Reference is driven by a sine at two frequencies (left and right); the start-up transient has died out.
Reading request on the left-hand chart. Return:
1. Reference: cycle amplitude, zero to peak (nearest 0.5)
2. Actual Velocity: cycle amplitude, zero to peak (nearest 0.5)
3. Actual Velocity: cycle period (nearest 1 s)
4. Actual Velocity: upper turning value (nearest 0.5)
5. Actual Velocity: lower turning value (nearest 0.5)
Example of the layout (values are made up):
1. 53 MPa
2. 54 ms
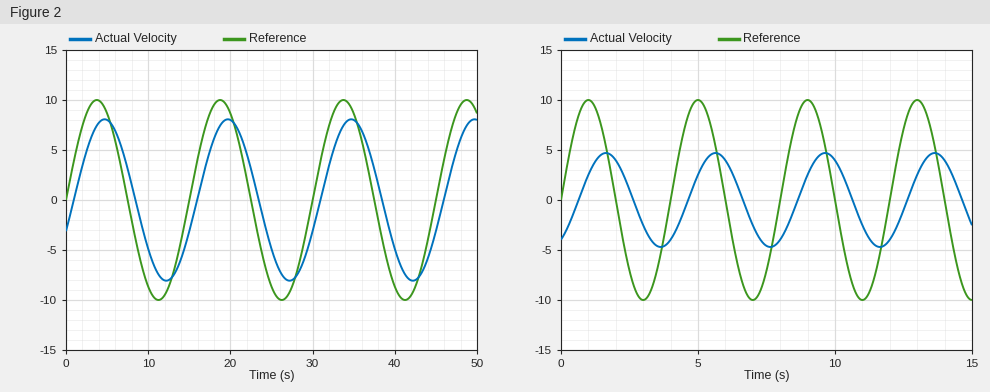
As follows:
1. 10.0
2. 8.0
3. 15 s
4. 8.0
5. -8.0
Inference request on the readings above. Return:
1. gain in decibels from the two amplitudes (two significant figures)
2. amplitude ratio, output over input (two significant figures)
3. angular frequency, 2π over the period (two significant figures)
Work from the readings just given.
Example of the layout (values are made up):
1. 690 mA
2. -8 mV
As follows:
1. -1.9 dB
2. 0.80
3. 0.42 rad/s
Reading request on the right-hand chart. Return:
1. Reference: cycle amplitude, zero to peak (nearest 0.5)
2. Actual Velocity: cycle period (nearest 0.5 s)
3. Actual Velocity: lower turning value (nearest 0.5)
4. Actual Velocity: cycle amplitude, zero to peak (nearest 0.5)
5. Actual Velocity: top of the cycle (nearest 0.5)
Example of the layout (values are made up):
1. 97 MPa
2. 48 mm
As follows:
1. 10.0
2. 4.0 s
3. -4.5
4. 4.5
5. 4.5
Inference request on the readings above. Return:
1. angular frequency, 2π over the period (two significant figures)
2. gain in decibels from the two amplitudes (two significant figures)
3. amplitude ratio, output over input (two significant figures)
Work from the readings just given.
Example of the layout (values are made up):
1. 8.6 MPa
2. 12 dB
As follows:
1. 1.6 rad/s
2. -6.9 dB
3. 0.45
